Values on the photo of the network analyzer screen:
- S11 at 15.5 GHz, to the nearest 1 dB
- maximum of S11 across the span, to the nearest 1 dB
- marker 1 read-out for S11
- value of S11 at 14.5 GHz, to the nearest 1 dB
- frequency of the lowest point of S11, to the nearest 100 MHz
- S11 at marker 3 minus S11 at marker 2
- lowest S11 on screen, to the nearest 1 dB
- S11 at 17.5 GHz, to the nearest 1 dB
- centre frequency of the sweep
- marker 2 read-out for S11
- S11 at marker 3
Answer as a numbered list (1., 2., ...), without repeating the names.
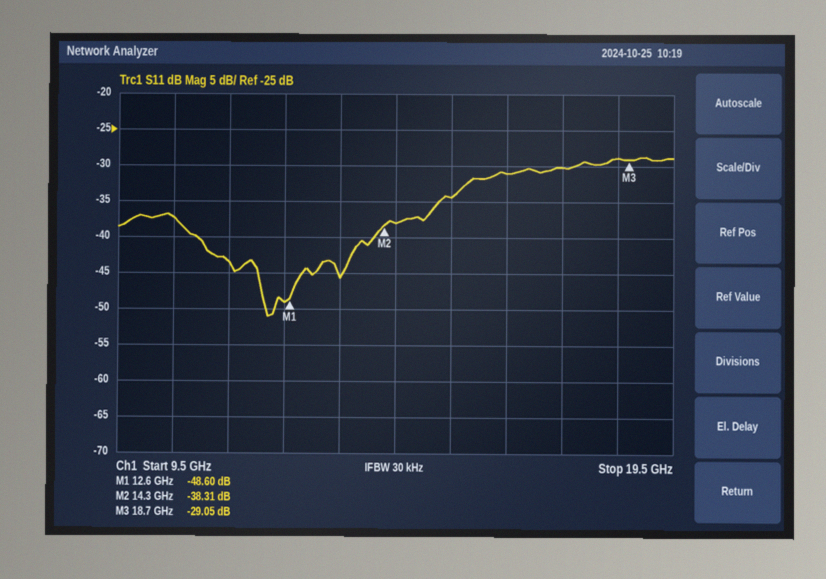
1. -34 dB
2. -29 dB
3. -48.60 dB
4. -38 dB
5. 12.2 GHz
6. 9.26 dB
7. -51 dB
8. -30 dB
9. 14.5 GHz
10. -38.31 dB
11. -29.05 dB
